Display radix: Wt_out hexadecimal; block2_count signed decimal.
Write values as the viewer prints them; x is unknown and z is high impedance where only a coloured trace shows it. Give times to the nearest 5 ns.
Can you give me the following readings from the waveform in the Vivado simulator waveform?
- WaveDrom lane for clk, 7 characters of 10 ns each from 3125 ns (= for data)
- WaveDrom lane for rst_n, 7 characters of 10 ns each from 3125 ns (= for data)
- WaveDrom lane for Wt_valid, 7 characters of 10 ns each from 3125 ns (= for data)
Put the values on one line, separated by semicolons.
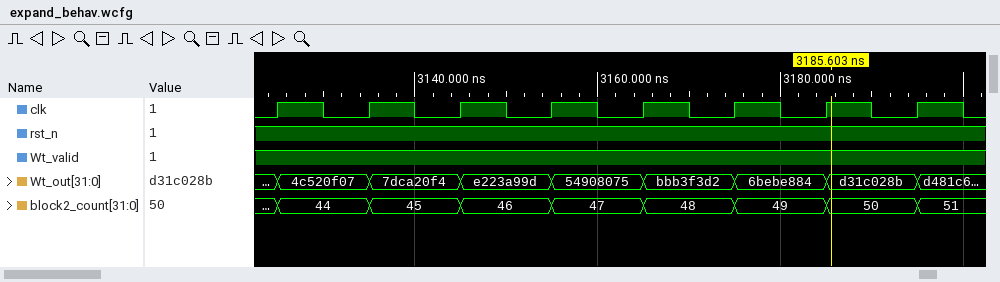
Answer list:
{name: 'clk', wave: 'p......'}; {name: 'rst_n', wave: '1......'}; {name: 'Wt_valid', wave: '1......'}
